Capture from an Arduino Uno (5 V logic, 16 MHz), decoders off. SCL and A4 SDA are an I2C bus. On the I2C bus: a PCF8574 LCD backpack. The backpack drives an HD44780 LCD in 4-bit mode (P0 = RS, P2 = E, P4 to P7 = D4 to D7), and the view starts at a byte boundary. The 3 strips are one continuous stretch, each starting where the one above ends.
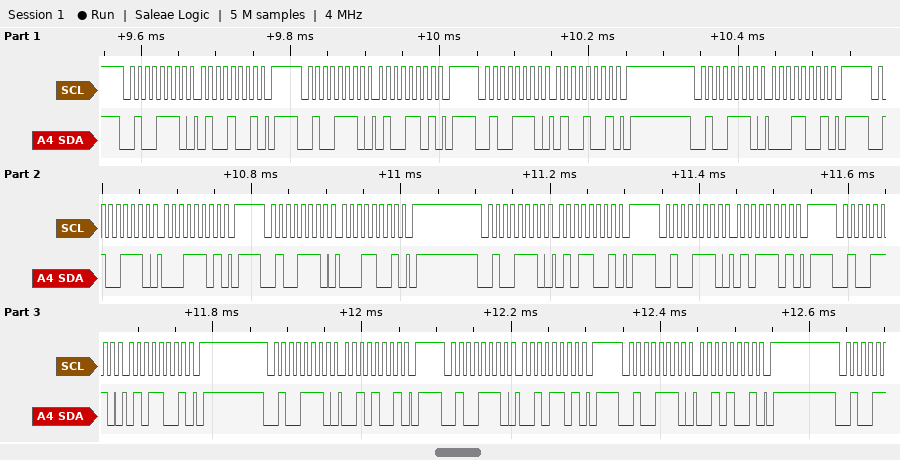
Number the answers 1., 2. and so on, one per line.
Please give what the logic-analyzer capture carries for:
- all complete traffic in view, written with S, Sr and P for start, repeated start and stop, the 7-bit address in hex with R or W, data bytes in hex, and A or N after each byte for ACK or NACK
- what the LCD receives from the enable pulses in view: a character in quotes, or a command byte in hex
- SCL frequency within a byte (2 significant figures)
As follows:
1. S 27W A 49 A P S 27W A 4D A P S 27W A 49 A P S 27W A 19 A P S 27W A 1D A P S 27W A 19 A P S 27W A 59 A P S 27W A 5D A P S 27W A 59 A P S 27W A 29 A P S 27W A 2D A P S 27W A 29 A P
2. 'A' 'R'
3. 100 kHz
